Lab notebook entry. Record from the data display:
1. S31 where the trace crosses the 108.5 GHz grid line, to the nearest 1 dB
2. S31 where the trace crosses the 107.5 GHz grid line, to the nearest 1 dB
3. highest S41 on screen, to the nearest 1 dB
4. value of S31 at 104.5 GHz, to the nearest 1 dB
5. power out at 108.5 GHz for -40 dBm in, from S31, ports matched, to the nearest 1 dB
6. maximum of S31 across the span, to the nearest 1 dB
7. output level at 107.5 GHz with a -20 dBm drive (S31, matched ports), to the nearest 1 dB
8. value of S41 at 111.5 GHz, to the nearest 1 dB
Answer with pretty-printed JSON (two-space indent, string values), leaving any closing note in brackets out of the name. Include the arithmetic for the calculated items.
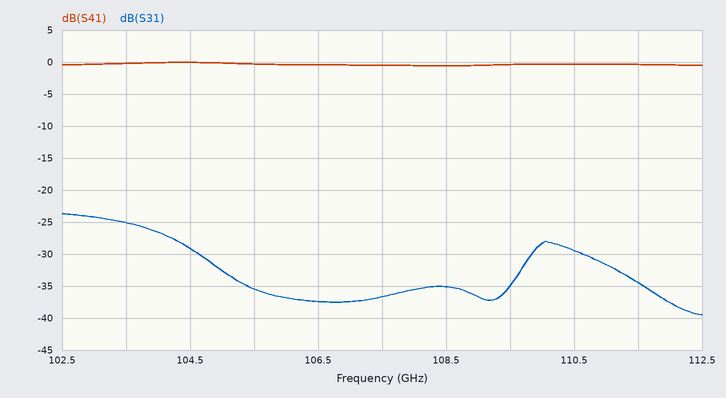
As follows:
{
  "S31 where the trace crosses the 108.5 GHz grid line, to the nearest 1 dB": "-35 dB",
  "S31 where the trace crosses the 107.5 GHz grid line, to the nearest 1 dB": "-37 dB",
  "highest S41 on screen, to the nearest 1 dB": "0 dB",
  "value of S31 at 104.5 GHz, to the nearest 1 dB": "-29 dB",
  "power out at 108.5 GHz for -40 dBm in, from S31, ports matched, to the nearest 1 dB": "-40 dBm + (-35 dB) = -75 dBm",
  "maximum of S31 across the span, to the nearest 1 dB": "-24 dB",
  "output level at 107.5 GHz with a -20 dBm drive (S31, matched ports), to the nearest 1 dB": "-20 dBm + (-37 dB) = -57 dBm",
  "value of S41 at 111.5 GHz, to the nearest 1 dB": "0 dB"
}
